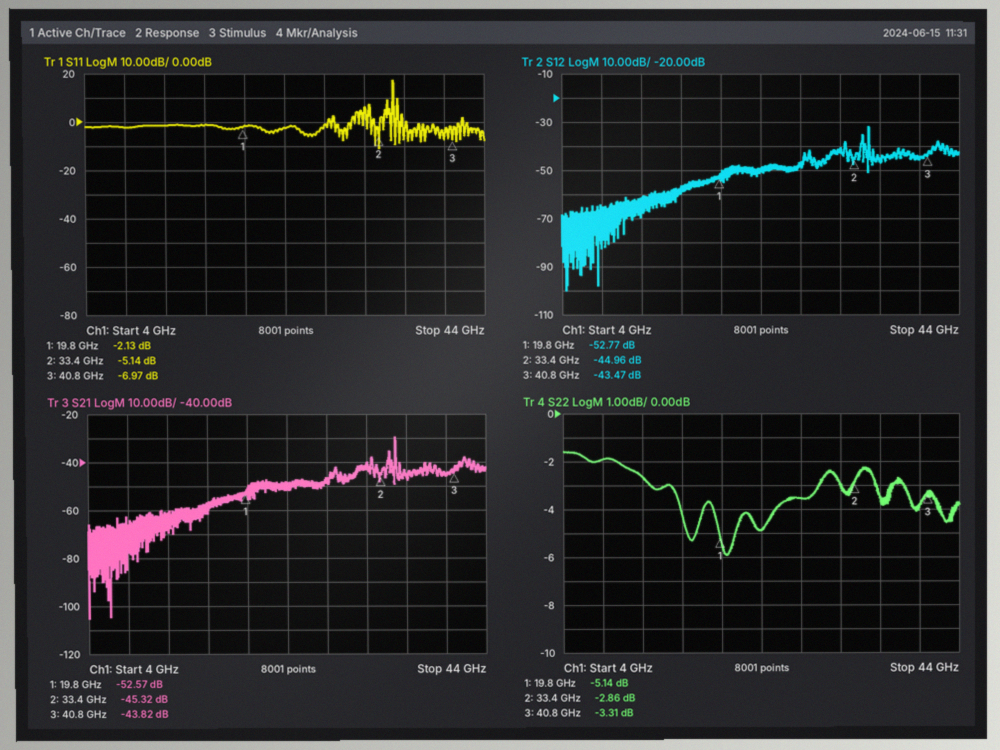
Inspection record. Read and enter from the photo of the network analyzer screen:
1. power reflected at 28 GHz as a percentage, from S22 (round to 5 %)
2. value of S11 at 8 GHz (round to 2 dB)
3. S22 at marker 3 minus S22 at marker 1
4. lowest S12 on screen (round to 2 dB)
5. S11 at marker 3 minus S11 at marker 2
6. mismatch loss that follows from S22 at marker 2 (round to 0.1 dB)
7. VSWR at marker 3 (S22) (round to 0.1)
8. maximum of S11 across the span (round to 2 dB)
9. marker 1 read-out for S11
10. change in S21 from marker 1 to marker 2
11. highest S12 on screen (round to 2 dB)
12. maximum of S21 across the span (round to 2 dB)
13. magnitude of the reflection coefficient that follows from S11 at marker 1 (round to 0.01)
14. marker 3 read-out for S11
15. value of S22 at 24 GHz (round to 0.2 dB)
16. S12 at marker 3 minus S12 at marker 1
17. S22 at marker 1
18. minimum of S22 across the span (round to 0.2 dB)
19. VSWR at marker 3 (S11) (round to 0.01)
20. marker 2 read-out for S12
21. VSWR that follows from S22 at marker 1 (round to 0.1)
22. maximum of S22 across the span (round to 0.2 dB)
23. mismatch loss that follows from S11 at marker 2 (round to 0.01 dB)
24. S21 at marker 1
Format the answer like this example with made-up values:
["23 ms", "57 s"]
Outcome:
["45 %", "-2 dB", "1.83 dB", "-100 dB", "-1.83 dB", "3.2 dB", "5.3", "18 dB", "-2.13 dB", "7.25 dB", "-32 dB", "-30 dB", "0.78", "-6.97 dB", "-4.8 dB", "9.30 dB", "-5.14 dB", "-6.0 dB", "2.62", "-44.96 dB", "3.5", "-1.6 dB", "1.59 dB", "-52.57 dB"]
